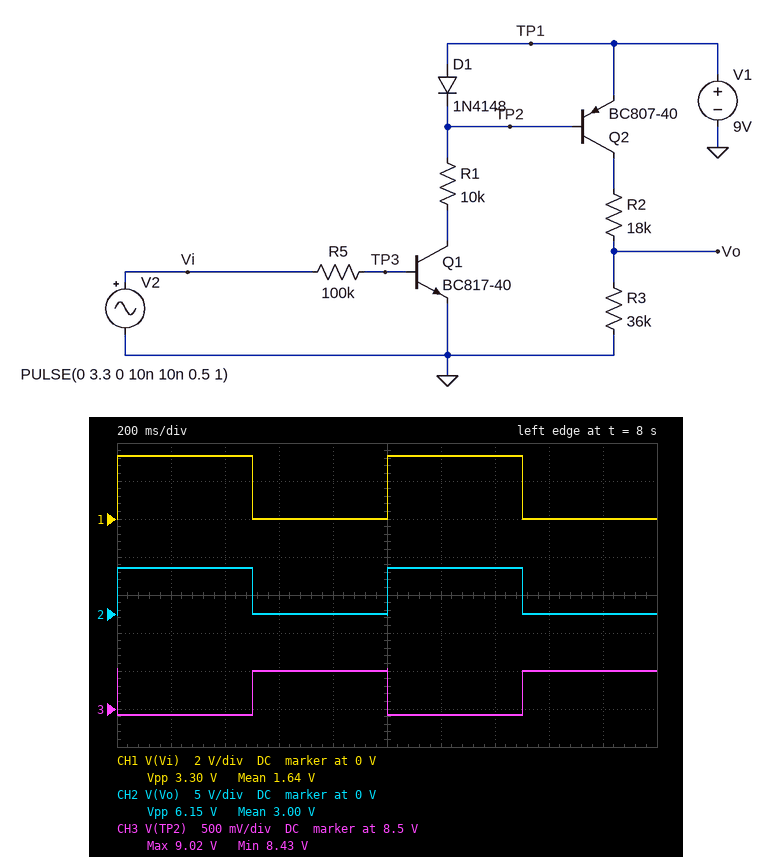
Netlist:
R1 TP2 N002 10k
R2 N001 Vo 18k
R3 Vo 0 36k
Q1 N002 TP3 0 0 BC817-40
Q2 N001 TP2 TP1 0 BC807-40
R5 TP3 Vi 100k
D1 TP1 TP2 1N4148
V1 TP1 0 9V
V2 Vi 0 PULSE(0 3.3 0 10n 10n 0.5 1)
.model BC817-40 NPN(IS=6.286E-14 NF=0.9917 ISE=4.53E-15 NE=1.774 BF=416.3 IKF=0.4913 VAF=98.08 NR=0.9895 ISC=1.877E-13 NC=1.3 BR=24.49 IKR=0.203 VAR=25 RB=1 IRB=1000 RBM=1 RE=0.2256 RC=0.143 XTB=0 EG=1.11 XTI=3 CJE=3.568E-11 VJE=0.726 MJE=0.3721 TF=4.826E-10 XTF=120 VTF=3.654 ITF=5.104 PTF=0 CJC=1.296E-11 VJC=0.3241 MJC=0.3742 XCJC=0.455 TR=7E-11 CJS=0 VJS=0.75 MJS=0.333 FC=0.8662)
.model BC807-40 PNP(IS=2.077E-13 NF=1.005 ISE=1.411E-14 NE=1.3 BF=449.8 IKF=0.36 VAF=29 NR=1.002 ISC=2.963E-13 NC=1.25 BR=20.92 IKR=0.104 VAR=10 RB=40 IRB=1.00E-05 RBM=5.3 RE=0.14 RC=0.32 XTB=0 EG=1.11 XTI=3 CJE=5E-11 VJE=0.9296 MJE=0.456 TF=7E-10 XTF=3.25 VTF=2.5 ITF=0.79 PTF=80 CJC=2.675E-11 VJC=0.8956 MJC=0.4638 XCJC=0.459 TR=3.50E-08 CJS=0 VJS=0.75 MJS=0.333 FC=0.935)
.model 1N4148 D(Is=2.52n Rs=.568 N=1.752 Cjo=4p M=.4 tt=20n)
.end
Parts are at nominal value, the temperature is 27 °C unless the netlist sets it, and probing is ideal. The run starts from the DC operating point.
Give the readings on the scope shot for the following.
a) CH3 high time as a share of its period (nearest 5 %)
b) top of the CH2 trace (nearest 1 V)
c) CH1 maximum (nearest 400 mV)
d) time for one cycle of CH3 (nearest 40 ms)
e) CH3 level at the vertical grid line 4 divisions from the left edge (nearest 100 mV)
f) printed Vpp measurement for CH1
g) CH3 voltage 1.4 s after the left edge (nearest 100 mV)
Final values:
50 %
6 V
3.2 V
1.00 s
9.0 V
3.30 V
8.4 V
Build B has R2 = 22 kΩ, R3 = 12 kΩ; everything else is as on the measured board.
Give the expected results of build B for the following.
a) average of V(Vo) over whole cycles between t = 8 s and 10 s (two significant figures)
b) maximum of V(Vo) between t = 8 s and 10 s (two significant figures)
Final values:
1.6 V
3.2 V
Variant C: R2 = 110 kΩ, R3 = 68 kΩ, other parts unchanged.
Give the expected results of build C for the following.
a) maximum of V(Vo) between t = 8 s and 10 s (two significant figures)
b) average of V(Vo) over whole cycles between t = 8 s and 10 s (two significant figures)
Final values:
3.4 V
1.7 V
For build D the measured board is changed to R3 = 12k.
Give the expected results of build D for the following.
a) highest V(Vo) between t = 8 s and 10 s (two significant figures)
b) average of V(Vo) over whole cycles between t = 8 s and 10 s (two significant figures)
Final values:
3.6 V
1.8 V
